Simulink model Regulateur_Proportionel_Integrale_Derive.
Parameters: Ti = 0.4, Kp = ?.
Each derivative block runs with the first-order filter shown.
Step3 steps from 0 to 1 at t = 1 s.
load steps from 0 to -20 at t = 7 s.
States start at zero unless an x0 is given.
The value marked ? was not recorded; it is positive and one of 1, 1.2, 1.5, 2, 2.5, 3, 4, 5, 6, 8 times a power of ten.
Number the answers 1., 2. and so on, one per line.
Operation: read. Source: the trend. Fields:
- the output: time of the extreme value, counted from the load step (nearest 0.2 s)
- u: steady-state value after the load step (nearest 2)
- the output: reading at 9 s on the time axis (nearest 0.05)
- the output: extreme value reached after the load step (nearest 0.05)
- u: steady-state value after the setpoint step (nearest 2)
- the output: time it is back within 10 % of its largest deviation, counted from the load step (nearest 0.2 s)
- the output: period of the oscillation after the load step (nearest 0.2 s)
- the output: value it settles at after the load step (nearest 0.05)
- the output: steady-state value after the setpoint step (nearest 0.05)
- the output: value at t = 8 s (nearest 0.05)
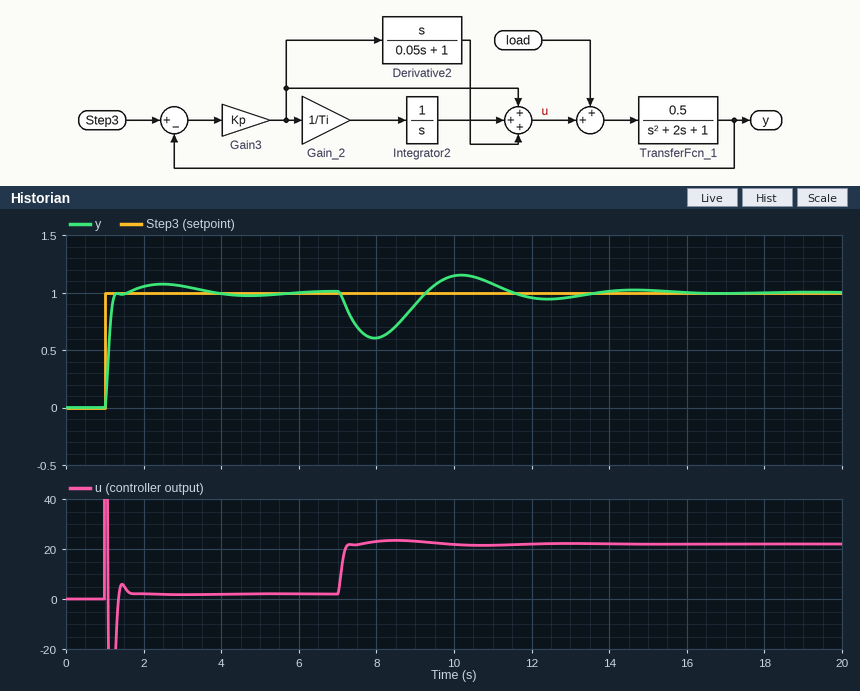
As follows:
1. 1.0 s
2. 22
3. 0.90
4. 0.60
5. 2
6. 6.0 s
7. 4.4 s
8. 1.00
9. 1.00
10. 0.60
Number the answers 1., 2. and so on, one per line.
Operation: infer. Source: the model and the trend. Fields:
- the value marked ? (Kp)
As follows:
1. 20
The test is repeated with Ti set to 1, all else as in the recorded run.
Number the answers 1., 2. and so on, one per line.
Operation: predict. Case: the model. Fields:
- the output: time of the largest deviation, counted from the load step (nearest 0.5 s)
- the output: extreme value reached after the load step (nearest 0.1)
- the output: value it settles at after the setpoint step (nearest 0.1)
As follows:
1. 1.5 s
2. 0.5
3. 1.0
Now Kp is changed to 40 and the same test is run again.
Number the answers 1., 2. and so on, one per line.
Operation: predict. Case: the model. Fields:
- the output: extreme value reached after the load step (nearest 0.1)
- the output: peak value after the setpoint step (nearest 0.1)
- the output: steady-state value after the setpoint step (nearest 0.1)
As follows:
1. 0.8
2. 1.1
3. 1.0
